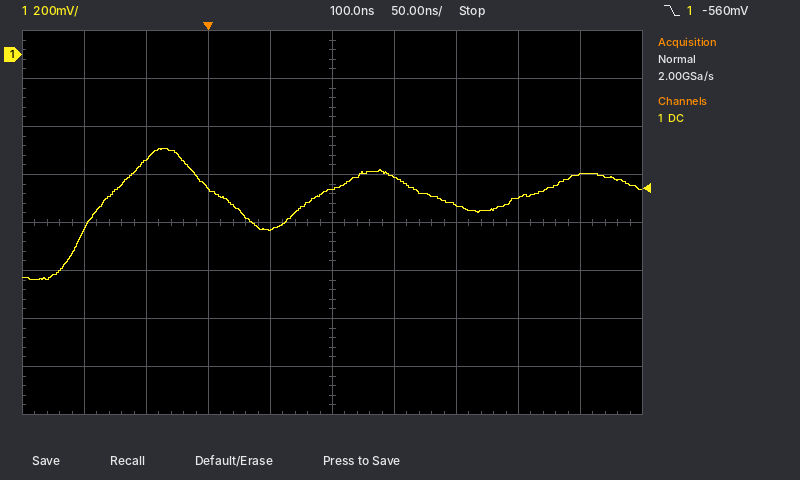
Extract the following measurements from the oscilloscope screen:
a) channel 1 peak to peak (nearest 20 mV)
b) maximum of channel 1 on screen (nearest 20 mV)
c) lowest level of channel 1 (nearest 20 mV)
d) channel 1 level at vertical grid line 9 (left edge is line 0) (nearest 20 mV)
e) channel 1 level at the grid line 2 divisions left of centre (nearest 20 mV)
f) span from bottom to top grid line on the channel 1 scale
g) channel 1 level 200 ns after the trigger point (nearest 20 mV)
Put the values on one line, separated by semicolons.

540 mV; -400 mV; -940 mV; -500 mV; -560 mV; 1.6 V; -620 mV
